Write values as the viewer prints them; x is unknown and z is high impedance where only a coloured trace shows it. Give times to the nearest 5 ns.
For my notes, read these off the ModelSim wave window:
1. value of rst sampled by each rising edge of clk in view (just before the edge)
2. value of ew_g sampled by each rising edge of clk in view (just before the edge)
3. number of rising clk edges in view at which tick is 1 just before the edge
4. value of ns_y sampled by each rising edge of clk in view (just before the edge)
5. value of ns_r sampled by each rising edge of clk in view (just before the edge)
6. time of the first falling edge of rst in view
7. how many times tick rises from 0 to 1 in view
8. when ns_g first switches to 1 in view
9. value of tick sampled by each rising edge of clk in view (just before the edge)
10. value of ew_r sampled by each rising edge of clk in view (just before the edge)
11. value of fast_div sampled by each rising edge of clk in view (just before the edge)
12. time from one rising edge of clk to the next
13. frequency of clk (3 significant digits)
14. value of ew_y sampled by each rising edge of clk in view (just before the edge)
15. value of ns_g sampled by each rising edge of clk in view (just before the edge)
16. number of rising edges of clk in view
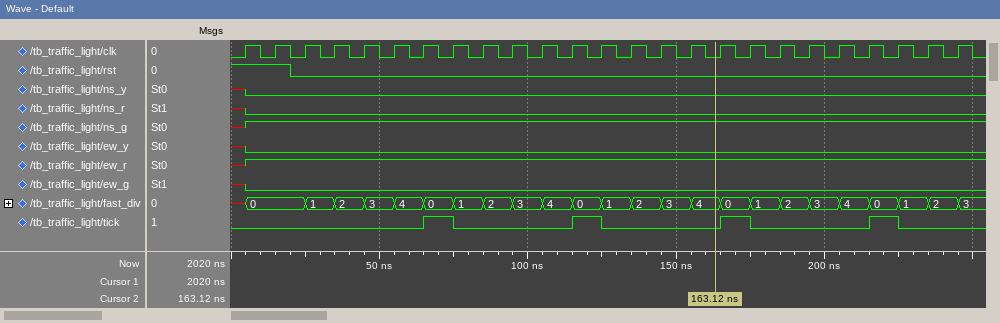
1 1 0 0 0 0 0 0 0 0 0 0 0 0 0 0 0 0 0 0 0 0 0 0 0
x 0 0 0 0 0 0 0 0 0 0 0 0 0 0 0 0 0 0 0 0 0 0 0 0
4
x 0 0 0 0 0 0 0 0 0 0 0 0 0 0 0 0 0 0 0 0 0 0 0 0
x 0 0 0 0 0 0 0 0 0 0 0 0 0 0 0 0 0 0 0 0 0 0 0 0
20 ns
4
5 ns
0 0 0 0 0 0 0 1 0 0 0 0 1 0 0 0 0 1 0 0 0 0 1 0 0
x 1 1 1 1 1 1 1 1 1 1 1 1 1 1 1 1 1 1 1 1 1 1 1 1
x, 0, 0, 1, 2, 3, 4, 0, 1, 2, 3, 4, 0, 1, 2, 3, 4, 0, 1, 2, 3, 4, 0, 1, 2
10 ns
100 MHz
x 0 0 0 0 0 0 0 0 0 0 0 0 0 0 0 0 0 0 0 0 0 0 0 0
x 1 1 1 1 1 1 1 1 1 1 1 1 1 1 1 1 1 1 1 1 1 1 1 1
25
